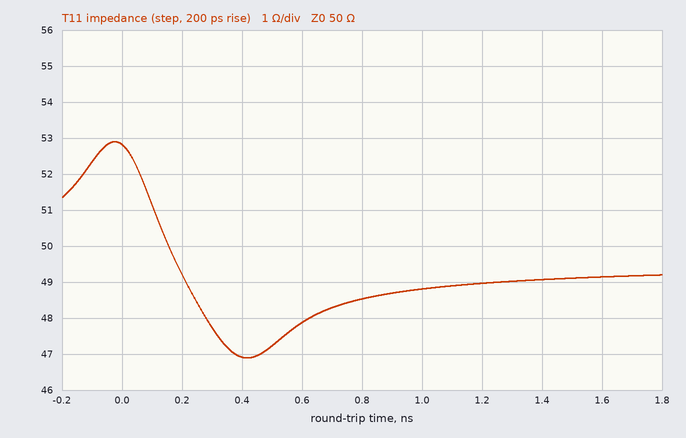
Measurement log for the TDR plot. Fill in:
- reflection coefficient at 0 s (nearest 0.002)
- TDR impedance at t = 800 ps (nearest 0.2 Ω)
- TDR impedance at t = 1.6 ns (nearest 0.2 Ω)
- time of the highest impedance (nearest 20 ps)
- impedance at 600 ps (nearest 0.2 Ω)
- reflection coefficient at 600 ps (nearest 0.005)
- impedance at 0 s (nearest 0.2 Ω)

+0.028
48.6 Ω
49.2 Ω
-20 ps
47.8 Ω
-0.020
52.8 Ω
